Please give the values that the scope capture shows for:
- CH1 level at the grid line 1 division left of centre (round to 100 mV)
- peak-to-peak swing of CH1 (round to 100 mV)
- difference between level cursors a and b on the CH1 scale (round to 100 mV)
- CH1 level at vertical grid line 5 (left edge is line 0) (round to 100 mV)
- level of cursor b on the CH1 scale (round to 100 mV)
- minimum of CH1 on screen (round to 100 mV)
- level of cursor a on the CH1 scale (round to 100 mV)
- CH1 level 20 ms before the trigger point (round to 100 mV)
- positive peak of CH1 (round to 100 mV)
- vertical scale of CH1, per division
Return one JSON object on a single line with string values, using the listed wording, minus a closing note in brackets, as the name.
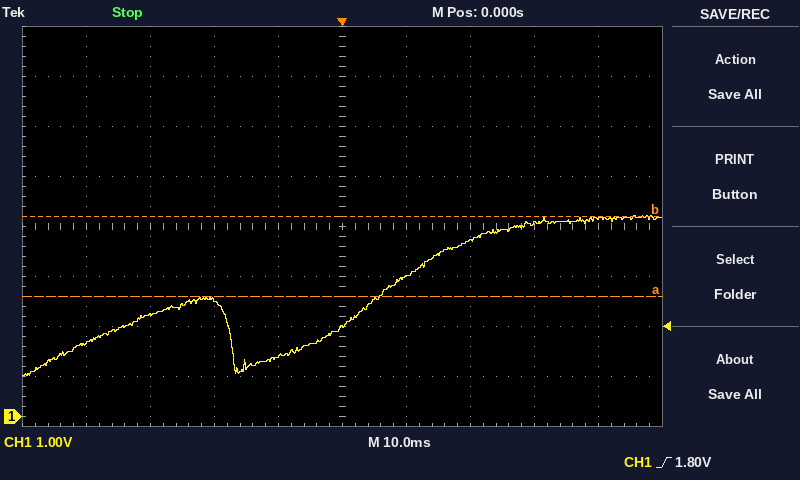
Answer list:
{"CH1 level at the grid line 1 division left of centre": "1.2 V", "peak-to-peak swing of CH1": "3.2 V", "difference between level cursors a and b on the CH1 scale": "1.6 V", "CH1 level at vertical grid line 5 (left edge is line 0)": "1.8 V", "level of cursor b on the CH1 scale": "4.0 V", "minimum of CH1 on screen": "800 mV", "level of cursor a on the CH1 scale": "2.4 V", "CH1 level 20 ms before the trigger point": "2.3 V", "positive peak of CH1": "4.0 V", "vertical scale of CH1, per division": "1 V"}
